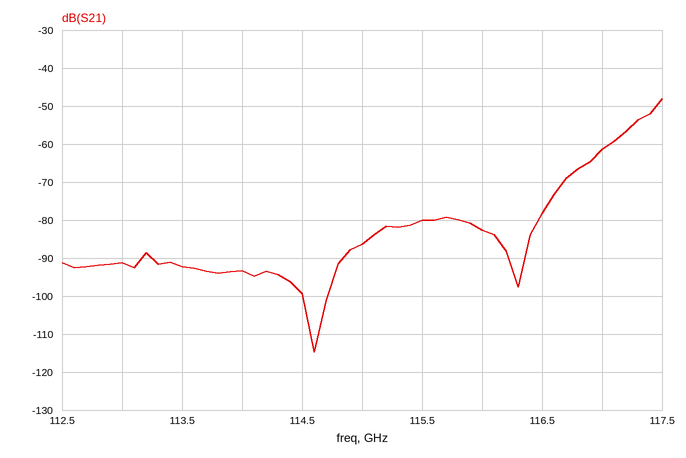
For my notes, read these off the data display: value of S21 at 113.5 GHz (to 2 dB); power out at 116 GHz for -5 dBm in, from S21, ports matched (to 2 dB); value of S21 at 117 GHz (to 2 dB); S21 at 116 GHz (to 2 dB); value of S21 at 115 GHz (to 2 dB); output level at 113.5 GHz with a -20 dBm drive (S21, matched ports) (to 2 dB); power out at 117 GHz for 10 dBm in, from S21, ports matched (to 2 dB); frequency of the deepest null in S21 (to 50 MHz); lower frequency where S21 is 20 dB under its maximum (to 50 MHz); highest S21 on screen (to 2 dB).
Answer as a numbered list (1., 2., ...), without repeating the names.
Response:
1. -92 dB
2. -88 dBm
3. -62 dB
4. -82 dB
5. -86 dB
6. -112 dBm
7. -52 dBm
8. 114.60 GHz
9. 116.75 GHz
10. -48 dB
